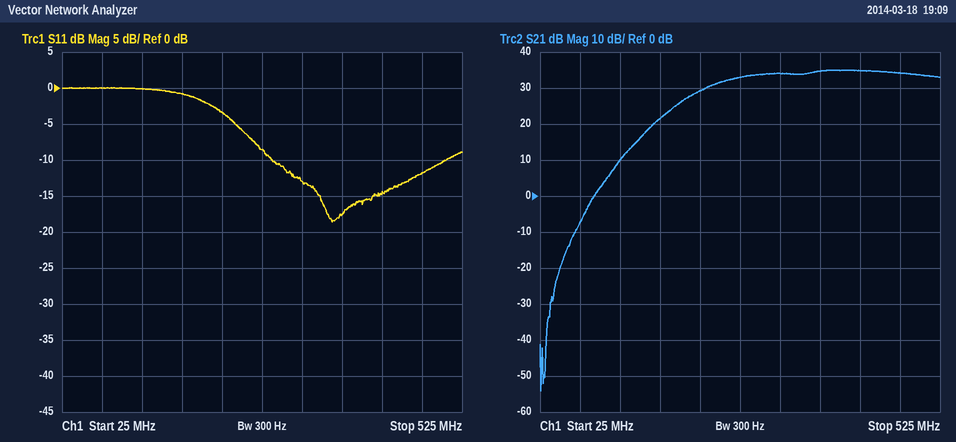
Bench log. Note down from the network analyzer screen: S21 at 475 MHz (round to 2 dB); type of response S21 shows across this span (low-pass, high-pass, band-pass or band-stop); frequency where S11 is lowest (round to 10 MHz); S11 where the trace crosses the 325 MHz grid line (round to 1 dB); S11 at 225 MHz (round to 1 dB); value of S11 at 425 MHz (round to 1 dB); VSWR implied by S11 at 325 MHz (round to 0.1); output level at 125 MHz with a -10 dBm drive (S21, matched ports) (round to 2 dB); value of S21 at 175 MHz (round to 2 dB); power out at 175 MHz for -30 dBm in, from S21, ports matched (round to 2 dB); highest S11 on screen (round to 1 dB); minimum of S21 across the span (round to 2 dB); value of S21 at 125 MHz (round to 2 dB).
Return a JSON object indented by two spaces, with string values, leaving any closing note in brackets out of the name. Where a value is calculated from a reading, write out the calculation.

{
  "S21 at 475 MHz": "34 dB",
  "type of response S21 shows across this span": "high-pass",
  "frequency where S11 is lowest": "360 MHz",
  "S11 where the trace crosses the 325 MHz grid line": "-13 dB",
  "S11 at 225 MHz": "-3 dB",
  "value of S11 at 425 MHz": "-15 dB",
  "VSWR implied by S11 at 325 MHz": "|Γ| = 10^(-13/20) = 0.2239; VSWR = (1 + 0.2239)/(1 − 0.2239) ≈ 1.6",
  "output level at 125 MHz with a -10 dBm drive (S21, matched ports)": "-10 dBm + (10 dB) = 0 dBm",
  "value of S21 at 175 MHz": "22 dB",
  "power out at 175 MHz for -30 dBm in, from S21, ports matched": "-30 dBm + (22 dB) = -8 dBm",
  "highest S11 on screen": "0 dB",
  "minimum of S21 across the span": "-54 dB",
  "value of S21 at 125 MHz": "10 dB"
}
